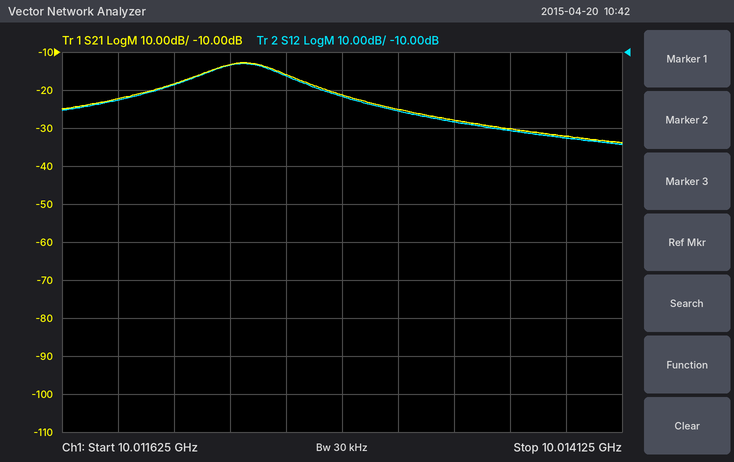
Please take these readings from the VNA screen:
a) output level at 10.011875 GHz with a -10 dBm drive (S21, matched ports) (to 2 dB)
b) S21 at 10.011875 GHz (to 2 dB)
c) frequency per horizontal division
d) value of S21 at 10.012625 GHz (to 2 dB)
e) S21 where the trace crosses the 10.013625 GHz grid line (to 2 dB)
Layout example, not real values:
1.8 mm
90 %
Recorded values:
-32 dBm
-22 dB
250 kHz
-16 dB
-30 dB
